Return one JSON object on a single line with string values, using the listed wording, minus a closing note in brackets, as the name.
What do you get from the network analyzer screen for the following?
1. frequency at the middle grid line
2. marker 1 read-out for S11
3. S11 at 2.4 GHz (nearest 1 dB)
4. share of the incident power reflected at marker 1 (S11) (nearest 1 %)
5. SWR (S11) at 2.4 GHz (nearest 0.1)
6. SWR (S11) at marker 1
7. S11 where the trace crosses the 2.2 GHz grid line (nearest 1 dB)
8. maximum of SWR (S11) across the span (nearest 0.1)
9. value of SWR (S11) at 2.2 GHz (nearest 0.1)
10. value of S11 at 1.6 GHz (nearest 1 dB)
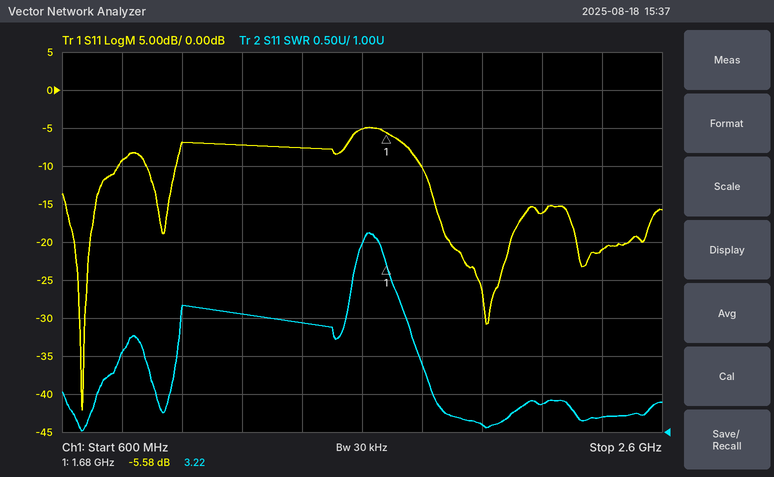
{"frequency at the middle grid line": "1.6 GHz", "marker 1 read-out for S11": "-5.58 dB", "S11 at 2.4 GHz": "-21 dB", "share of the incident power reflected at marker 1 (S11)": "28 %", "SWR (S11) at 2.4 GHz": "1.2", "SWR (S11) at marker 1": "3.22", "S11 where the trace crosses the 2.2 GHz grid line": "-16 dB", "maximum of SWR (S11) across the span": "3.6", "value of SWR (S11) at 2.2 GHz": "1.4", "value of S11 at 1.6 GHz": "-5 dB"}
